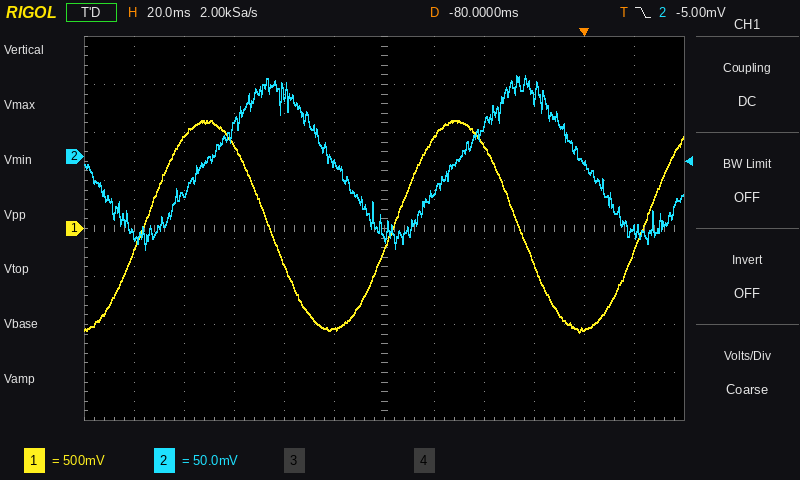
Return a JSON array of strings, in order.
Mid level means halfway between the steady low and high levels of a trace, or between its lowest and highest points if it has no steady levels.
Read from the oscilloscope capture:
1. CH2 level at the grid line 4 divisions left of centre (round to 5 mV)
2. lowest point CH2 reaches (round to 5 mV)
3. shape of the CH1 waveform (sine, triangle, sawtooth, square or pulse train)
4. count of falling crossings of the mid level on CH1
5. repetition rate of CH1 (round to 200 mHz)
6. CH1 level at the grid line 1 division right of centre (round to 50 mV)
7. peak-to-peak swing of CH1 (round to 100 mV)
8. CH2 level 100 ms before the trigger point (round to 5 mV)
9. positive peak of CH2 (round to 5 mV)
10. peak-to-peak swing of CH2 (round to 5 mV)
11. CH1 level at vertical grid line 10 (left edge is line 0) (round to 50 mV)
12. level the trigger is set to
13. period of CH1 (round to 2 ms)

["-40 mV", "-95 mV", "sine", "2", "10.0 Hz", "950 mV", "2.20 V", "-5 mV", "85 mV", "180 mV", "-1.05 V", "-5.00 mV", "100 ms"]
